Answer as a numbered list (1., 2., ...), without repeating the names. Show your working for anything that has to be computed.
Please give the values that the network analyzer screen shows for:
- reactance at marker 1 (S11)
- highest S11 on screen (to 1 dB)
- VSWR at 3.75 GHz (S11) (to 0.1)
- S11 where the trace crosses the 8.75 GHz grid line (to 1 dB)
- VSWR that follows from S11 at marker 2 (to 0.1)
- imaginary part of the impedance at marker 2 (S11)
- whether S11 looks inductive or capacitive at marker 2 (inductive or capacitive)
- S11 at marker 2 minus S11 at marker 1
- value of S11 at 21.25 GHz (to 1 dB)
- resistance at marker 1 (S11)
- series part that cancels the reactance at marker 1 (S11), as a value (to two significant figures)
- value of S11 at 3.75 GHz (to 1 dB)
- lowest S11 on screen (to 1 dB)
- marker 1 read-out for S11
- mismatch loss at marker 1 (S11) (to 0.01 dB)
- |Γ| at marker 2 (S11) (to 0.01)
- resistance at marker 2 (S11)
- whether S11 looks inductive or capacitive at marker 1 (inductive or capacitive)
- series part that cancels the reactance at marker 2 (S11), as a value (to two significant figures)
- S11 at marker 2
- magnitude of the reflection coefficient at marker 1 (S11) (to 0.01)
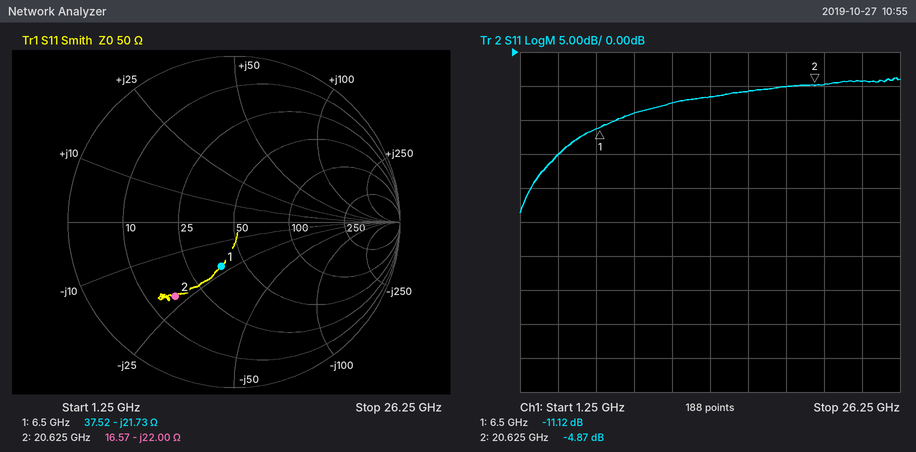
1. -21.73 Ω
2. -4 dB
3. |Γ| = 10^(-15/20) = 0.1778; VSWR = (1 + 0.1778)/(1 − 0.1778) ≈ 1.4
4. -9 dB
5. (1 + 0.5708)/(1 − 0.5708) ≈ 3.7
6. -22.00 Ω
7. capacitive
8. -4.87 − (-11.12) = 6.25 dB
9. -5 dB
10. 37.52 Ω
11. L = 21.73 Ω/(2π × 6.5 GHz) ≈ 532 pH, so 530 pH to two significant figures
12. -15 dB
13. -24 dB
14. -11.12 dB
15. −10 log10(1 − 10^(-11.12/10)) ≈ 0.35 dB
16. 0.57
17. 16.57 Ω
18. capacitive
19. L = 22 Ω/(2π × 20.625 GHz) ≈ 170 pH
20. -4.87 dB
21. 0.28
